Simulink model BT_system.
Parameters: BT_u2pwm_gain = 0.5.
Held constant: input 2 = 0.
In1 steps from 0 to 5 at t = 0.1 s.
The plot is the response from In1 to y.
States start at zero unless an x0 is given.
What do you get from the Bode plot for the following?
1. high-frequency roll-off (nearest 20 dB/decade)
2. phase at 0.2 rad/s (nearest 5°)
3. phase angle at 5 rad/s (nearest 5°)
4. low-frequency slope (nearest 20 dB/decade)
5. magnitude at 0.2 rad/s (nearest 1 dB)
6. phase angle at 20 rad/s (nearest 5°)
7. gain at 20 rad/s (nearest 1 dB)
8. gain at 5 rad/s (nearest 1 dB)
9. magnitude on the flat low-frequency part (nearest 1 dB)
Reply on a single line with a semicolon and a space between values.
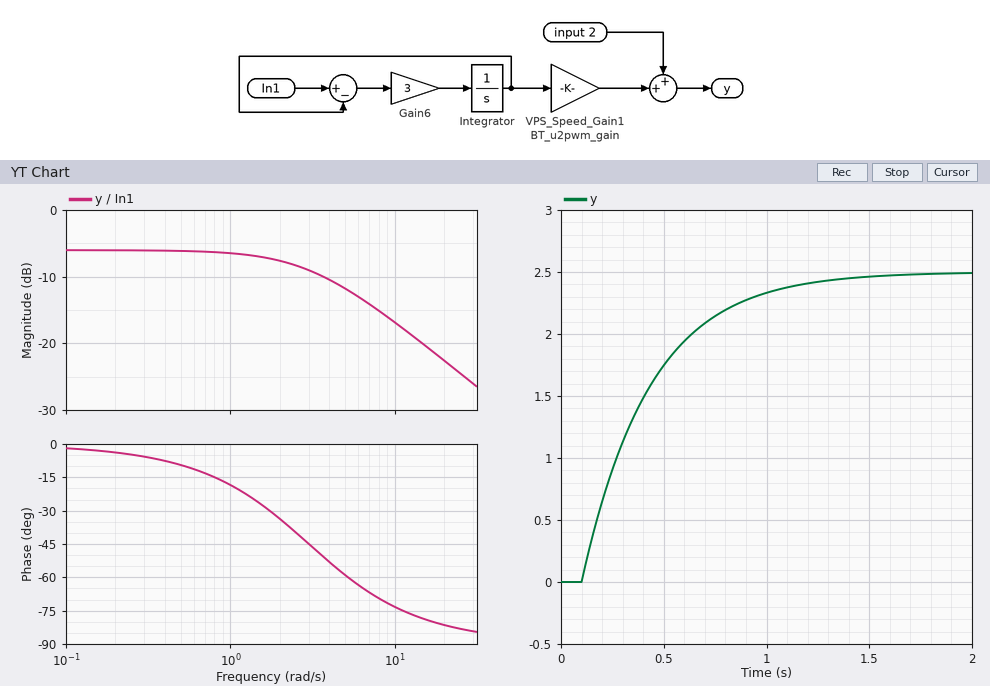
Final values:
-20 dB/decade; -5°; -60°; 0 dB/decade; -6 dB; -80°; -23 dB; -12 dB; -6 dB
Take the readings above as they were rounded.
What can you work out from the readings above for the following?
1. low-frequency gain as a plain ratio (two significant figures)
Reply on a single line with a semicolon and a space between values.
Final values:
0.50
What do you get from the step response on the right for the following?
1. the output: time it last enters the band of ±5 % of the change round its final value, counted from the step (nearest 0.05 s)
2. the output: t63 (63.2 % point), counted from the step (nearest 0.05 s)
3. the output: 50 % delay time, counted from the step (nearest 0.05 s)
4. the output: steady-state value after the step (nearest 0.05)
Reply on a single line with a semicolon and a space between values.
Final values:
1.00 s; 0.35 s; 0.25 s; 2.50
